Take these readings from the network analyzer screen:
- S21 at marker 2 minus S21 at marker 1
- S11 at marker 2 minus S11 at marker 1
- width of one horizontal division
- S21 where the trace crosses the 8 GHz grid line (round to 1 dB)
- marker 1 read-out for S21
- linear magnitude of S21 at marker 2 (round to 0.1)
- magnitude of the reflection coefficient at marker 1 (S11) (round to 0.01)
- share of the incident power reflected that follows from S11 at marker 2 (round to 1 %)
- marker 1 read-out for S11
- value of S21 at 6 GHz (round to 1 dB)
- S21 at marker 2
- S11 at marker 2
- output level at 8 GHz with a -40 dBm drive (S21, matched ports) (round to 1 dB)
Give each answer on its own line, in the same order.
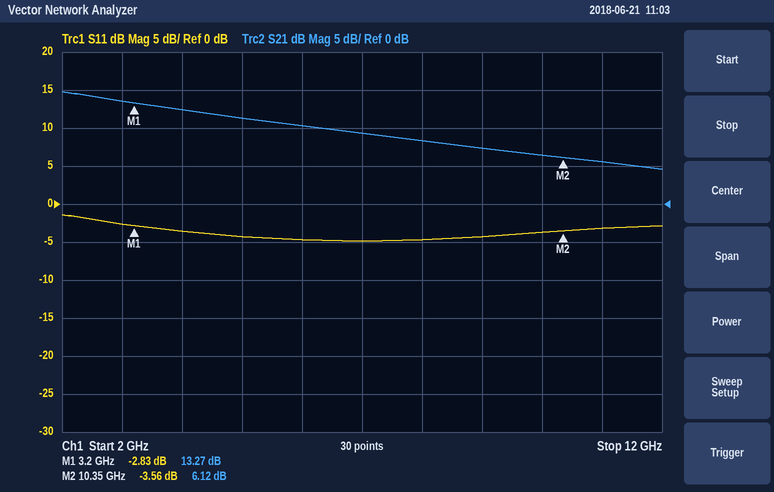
-7.15 dB
-0.73 dB
1 GHz
8 dB
13.27 dB
2.0
0.72
44 %
-2.83 dB
10 dB
6.12 dB
-3.56 dB
-32 dBm
